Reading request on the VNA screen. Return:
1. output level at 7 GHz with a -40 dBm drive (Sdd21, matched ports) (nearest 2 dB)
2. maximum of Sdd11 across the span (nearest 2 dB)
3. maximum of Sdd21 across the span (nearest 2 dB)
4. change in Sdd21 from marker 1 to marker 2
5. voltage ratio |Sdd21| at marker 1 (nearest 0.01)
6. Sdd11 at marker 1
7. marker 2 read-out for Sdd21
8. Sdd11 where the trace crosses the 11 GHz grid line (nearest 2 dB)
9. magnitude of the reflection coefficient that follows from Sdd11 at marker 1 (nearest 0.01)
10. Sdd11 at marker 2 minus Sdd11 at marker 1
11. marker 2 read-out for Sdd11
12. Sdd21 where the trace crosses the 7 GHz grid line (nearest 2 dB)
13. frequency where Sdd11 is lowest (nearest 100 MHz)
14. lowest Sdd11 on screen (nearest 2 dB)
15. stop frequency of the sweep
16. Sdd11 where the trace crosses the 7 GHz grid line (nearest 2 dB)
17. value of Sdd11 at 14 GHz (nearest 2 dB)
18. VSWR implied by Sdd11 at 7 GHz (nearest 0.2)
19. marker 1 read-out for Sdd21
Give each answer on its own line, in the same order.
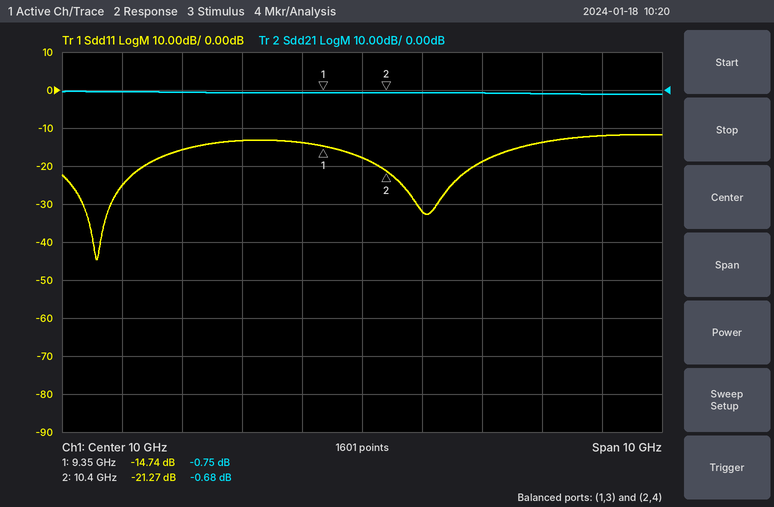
-40 dBm
-12 dB
0 dB
0.07 dB
0.92
-14.74 dB
-0.68 dB
-32 dB
0.18
-6.53 dB
-21.27 dB
0 dB
5.6 GHz
-44 dB
15 GHz
-16 dB
-12 dB
1.4
-0.75 dB
